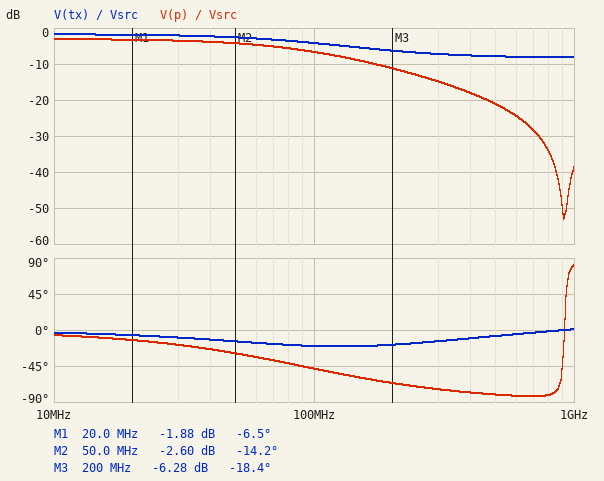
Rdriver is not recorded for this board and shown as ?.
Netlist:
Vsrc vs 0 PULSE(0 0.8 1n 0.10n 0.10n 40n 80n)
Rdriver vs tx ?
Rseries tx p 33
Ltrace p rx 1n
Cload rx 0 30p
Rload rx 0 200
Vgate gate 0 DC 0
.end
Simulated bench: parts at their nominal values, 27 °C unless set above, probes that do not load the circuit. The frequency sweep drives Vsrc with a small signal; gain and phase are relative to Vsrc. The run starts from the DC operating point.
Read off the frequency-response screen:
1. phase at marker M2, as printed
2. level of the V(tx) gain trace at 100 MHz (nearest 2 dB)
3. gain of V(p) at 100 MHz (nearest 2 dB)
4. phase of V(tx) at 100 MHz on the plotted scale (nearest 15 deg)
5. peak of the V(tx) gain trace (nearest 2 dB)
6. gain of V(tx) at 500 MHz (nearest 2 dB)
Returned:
-14.2 deg
-4 dB
-6 dB
-15 deg
-2 dB
-8 dB
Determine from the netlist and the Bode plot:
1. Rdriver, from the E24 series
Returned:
51 Ω
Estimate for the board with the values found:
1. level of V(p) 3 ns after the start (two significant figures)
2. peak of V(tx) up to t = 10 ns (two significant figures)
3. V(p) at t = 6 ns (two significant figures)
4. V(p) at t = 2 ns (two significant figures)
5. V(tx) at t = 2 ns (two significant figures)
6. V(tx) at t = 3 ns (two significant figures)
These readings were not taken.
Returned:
370 mV
650 mV
530 mV
230 mV
450 mV
540 mV
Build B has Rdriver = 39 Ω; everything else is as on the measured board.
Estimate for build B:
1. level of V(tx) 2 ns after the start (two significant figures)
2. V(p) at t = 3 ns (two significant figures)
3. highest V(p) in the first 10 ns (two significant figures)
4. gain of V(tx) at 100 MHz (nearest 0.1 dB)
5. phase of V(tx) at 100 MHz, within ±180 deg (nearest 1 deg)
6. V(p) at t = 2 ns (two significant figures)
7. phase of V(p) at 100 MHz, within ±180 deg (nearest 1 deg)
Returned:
510 mV
410 mV
590 mV
-3.3 dB
-17 deg
260 mV
-45 deg
